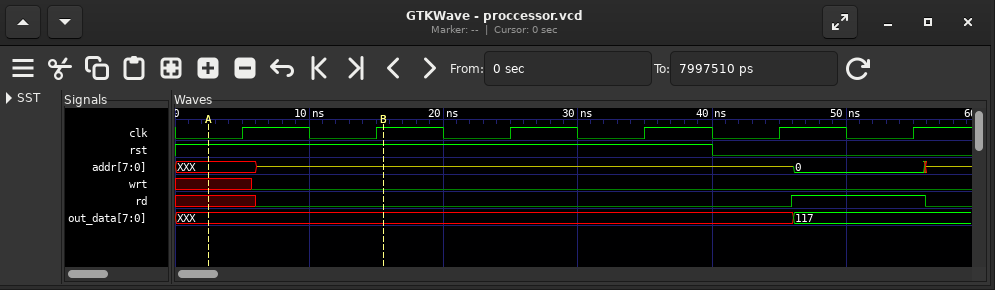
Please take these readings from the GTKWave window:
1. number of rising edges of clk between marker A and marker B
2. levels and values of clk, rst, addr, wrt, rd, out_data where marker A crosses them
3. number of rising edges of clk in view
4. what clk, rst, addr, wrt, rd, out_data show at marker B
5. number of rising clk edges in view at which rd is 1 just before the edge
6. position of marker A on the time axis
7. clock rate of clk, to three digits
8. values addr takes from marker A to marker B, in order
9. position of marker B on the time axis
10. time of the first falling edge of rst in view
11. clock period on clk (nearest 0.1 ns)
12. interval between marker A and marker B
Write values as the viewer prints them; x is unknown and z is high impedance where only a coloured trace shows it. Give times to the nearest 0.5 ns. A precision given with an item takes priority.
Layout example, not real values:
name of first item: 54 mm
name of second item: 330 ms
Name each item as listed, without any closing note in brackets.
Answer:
number of rising edges of clk between marker A and marker B: 2
levels and values of clk, rst, addr, wrt, rd, out_data where marker A crosses them: clk=0, rst=1, addr=XXX, wrt=x, rd=x, out_data=XXX
number of rising edges of clk in view: 6
what clk, rst, addr, wrt, rd, out_data show at marker B: clk=1, rst=1, addr=z, wrt=0, rd=0, out_data=XXX
number of rising clk edges in view at which rd is 1 just before the edge: 1
position of marker A on the time axis: 2.5 ns
clock rate of clk, to three digits: 100 MHz
values addr takes from marker A to marker B, in order: XXX, z
position of marker B on the time axis: 15.5 ns
time of the first falling edge of rst in view: 40 ns
clock period on clk: 10 ns
interval between marker A and marker B: 13 ns
